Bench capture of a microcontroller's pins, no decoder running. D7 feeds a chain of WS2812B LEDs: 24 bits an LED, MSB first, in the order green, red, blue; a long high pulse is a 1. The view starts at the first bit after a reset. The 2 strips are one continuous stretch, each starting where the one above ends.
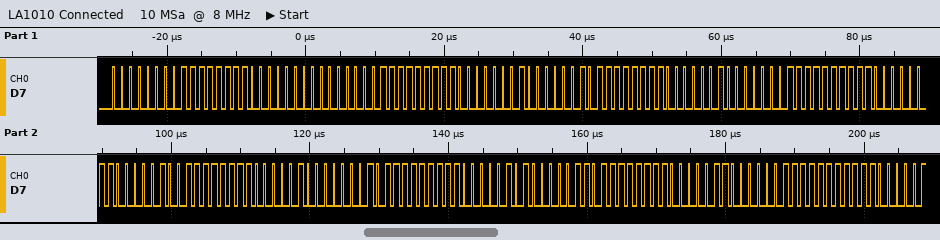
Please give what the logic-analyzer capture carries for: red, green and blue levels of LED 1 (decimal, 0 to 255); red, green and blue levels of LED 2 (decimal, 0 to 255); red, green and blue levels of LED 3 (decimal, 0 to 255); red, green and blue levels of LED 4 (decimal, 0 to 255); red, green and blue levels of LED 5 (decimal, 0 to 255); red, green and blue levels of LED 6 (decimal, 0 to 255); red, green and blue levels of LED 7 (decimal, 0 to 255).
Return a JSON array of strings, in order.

["255, 0, 0", "255, 1, 1", "255, 2, 2", "255, 3, 3", "255, 4, 4", "255, 5, 5", "255, 6, 6"]
